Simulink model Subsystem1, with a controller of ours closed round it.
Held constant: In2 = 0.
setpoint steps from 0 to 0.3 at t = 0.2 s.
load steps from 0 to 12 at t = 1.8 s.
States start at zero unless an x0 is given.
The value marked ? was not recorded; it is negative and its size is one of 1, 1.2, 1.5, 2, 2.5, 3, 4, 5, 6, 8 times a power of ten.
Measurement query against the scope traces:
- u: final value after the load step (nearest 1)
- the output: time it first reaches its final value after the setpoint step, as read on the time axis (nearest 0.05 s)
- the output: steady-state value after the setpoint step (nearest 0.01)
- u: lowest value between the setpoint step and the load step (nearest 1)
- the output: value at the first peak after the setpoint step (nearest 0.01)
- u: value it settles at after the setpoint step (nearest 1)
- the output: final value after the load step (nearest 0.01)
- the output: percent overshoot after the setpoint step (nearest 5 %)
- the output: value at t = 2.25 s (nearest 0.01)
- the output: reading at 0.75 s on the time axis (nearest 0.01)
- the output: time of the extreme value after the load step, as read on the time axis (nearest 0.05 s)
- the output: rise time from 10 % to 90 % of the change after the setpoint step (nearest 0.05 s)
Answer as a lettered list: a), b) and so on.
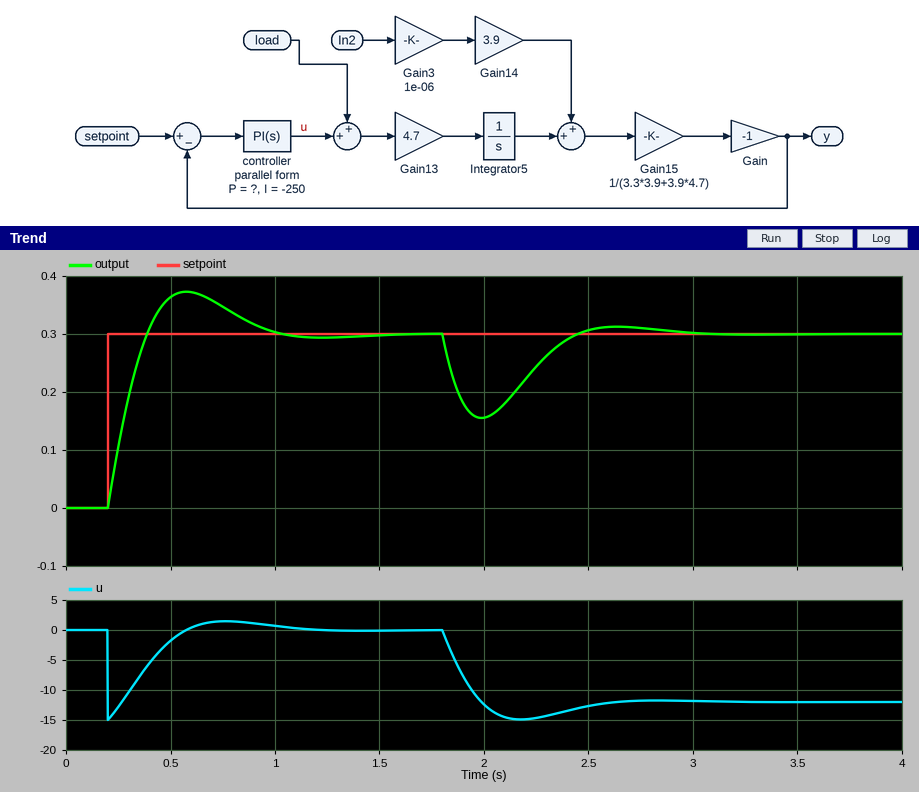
a) -12
b) 0.40 s
c) 0.30
d) -15
e) 0.37
f) 0
g) 0.30
h) 25 %
i) 0.24
j) 0.35
k) 2.00 s
l) 0.15 s
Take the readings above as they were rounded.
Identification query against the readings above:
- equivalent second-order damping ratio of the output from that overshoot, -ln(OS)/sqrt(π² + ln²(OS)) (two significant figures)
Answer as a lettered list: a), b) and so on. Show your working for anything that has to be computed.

a) ln(0.25) = -1.386; 1.386 / sqrt(9.870 + 1.922) = 0.40
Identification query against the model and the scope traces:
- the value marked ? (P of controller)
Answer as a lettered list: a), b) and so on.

a) -50
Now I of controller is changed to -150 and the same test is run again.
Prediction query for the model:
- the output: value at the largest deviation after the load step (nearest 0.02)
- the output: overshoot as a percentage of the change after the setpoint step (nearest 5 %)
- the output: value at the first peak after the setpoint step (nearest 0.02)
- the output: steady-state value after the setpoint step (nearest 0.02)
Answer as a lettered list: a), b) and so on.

a) 0.14
b) 20 %
c) 0.36
d) 0.30
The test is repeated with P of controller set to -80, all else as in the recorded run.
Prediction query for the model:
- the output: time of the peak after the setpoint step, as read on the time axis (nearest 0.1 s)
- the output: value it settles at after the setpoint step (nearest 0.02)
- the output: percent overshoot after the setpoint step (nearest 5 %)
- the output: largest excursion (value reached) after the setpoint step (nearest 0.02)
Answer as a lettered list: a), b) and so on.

a) 0.5 s
b) 0.30
c) 15 %
d) 0.34
